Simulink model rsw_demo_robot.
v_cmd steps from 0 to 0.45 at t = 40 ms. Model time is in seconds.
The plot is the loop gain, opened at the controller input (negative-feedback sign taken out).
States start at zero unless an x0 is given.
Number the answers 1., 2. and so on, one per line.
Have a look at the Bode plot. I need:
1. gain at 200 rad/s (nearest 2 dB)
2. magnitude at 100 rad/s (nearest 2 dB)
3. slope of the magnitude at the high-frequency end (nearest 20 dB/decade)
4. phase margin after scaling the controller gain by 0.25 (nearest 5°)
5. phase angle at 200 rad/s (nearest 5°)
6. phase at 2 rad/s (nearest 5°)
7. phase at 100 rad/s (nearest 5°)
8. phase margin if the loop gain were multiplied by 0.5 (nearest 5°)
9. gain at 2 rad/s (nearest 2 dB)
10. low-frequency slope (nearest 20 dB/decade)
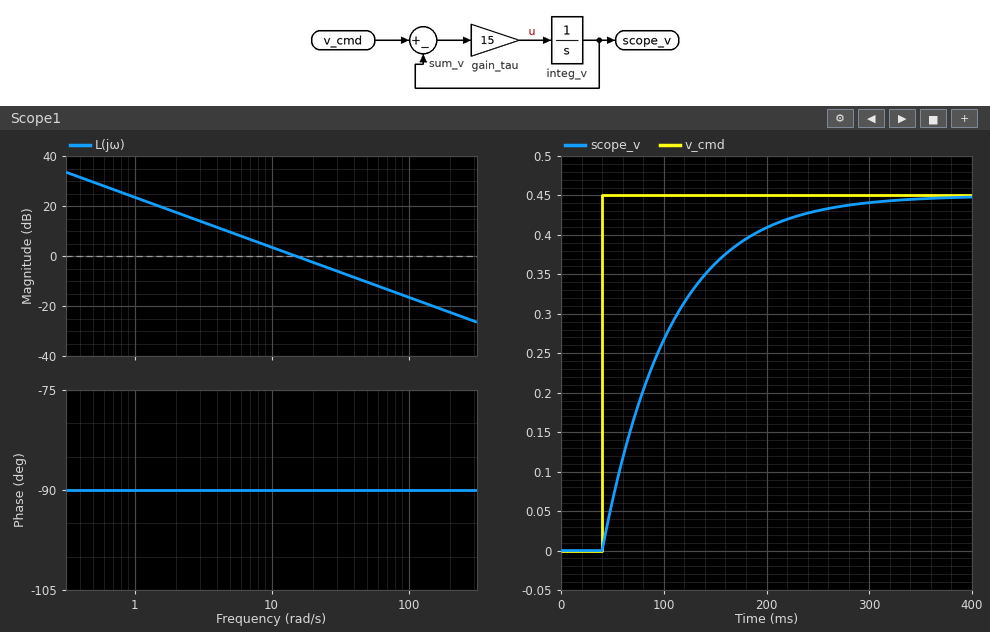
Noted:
1. -22 dB
2. -16 dB
3. -20 dB/decade
4. 90°
5. -90°
6. -90°
7. -90°
8. 90°
9. 18 dB
10. -20 dB/decade
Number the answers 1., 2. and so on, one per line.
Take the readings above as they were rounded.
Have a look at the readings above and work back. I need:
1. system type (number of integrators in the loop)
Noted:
1. 1
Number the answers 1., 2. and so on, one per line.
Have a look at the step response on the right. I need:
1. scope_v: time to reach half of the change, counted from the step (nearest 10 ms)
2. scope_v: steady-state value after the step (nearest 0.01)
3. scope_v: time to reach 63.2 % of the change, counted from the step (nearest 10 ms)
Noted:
1. 50 ms
2. 0.45
3. 70 ms
